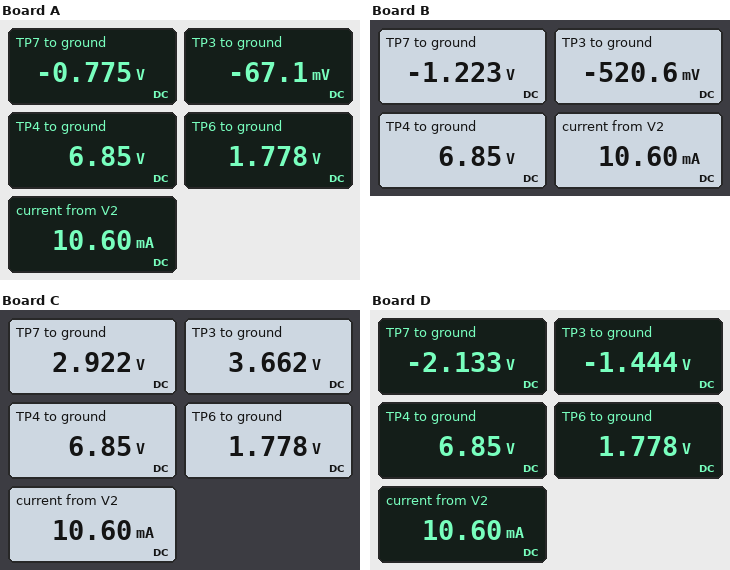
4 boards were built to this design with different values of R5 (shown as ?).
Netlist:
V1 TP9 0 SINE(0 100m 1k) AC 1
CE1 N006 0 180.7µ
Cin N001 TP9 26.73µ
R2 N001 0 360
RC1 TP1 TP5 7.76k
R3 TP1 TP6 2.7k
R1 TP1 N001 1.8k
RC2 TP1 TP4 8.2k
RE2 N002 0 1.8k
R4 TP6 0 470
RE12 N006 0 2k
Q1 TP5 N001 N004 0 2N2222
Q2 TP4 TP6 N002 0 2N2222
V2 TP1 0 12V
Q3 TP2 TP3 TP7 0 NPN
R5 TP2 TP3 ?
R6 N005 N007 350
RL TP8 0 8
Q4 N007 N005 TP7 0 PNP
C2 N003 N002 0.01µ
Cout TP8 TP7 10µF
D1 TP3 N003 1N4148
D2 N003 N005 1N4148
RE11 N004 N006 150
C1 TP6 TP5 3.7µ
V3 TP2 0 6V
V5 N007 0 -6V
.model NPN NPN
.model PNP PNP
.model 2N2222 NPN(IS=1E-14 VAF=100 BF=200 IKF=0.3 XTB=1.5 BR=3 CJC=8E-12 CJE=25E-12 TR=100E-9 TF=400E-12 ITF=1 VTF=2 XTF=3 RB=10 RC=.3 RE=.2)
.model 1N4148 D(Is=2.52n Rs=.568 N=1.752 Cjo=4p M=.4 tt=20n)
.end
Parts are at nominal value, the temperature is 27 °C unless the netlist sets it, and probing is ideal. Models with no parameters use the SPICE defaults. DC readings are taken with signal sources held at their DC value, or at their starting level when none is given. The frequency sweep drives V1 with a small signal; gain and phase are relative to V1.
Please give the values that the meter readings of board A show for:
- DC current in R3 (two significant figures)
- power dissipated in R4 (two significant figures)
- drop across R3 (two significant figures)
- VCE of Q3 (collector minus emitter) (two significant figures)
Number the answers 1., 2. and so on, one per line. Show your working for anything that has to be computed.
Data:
1. (12 V - 1.778 V) / 2.7 kΩ = 3.8 mA
2. (1.778 V)^2 / 470 Ω = 6.7 mW
3. 12 V - 1.778 V = 10 V
4. 6 V - (-775 mV) = 6.8 V
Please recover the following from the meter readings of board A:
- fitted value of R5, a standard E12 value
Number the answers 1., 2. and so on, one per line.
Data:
1. 470 Ω
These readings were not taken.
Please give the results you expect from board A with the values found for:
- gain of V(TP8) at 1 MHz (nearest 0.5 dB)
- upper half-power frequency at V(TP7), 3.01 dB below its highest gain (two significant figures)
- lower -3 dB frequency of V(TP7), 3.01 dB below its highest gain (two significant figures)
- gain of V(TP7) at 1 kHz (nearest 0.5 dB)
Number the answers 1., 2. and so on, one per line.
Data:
1. -24.0 dB
2. 2.0 MHz
3. 62 kHz
4. -52.5 dB
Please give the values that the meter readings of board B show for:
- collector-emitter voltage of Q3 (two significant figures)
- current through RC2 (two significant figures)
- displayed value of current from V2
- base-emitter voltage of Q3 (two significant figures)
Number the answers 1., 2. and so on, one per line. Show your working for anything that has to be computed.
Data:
1. 6 V - (-1.223 V) = 7.2 V
2. (12 V - 6.85 V) / 8.2 kΩ = 630 µA
3. 10.60 mA
4. -520.6 mV - (-1.223 V) = 700 mV
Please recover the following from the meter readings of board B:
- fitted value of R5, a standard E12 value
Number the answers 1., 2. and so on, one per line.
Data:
1. 560 Ω
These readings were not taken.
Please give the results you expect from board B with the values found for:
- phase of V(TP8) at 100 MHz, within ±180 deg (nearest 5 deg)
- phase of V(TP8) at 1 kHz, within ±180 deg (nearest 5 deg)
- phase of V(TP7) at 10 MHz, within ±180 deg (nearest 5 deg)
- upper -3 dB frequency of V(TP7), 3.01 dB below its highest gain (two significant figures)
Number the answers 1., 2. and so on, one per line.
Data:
1. 95 deg
2. -85 deg
3. 155 deg
4. 2.1 MHz
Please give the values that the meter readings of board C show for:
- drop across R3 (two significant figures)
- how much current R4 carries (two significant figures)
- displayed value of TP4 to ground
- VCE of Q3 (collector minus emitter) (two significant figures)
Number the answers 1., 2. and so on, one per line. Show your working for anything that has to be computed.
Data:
1. 12 V - 1.778 V = 10 V
2. (1.778 V) / 470 Ω = 3.8 mA
3. 6.85 V
4. 6 V - 2.922 V = 3.1 V
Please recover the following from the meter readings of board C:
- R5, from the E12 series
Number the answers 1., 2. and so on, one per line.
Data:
1. 100 Ω
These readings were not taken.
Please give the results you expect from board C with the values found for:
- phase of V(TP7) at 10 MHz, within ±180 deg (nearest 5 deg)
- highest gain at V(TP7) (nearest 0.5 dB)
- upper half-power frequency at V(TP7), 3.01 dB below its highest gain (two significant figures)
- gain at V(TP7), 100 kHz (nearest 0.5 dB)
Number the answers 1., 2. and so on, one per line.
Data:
1. 150 deg
2. -15.5 dB
3. 1.3 MHz
4. -19.0 dB
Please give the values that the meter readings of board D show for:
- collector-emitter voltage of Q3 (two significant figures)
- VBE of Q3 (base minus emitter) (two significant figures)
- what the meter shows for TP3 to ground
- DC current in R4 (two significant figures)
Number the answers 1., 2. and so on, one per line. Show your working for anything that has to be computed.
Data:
1. 6 V - (-2.133 V) = 8.1 V
2. -1.444 V - (-2.133 V) = 690 mV
3. -1.444 V
4. (1.778 V) / 470 Ω = 3.8 mA
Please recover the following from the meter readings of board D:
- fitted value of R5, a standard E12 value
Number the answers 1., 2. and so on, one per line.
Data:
1. 820 Ω
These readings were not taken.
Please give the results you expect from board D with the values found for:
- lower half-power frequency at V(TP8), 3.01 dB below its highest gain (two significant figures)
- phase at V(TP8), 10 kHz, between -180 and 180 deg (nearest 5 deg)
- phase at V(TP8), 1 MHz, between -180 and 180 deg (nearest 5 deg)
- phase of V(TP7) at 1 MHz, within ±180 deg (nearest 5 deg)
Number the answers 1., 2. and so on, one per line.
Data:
1. 53 kHz
2. -100 deg
3. 165 deg
4. 165 deg
